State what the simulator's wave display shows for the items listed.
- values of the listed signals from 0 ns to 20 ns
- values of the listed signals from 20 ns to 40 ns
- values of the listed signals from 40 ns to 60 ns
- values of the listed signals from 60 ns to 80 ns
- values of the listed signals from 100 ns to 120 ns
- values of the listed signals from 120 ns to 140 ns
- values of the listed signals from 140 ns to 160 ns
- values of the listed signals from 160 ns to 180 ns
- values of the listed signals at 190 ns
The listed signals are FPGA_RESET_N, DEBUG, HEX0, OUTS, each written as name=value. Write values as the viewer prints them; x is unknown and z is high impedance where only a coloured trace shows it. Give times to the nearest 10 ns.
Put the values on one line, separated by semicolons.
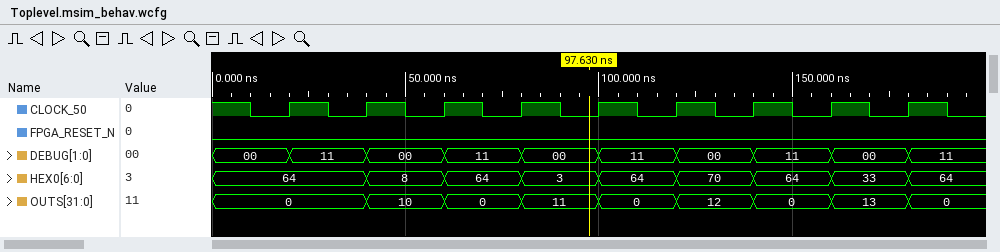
FPGA_RESET_N=0, DEBUG=00, HEX0=64, OUTS=0; FPGA_RESET_N=0, DEBUG=11, HEX0=64, OUTS=0; FPGA_RESET_N=0, DEBUG=00, HEX0=8, OUTS=10; FPGA_RESET_N=0, DEBUG=11, HEX0=64, OUTS=0; FPGA_RESET_N=0, DEBUG=11, HEX0=64, OUTS=0; FPGA_RESET_N=0, DEBUG=00, HEX0=70, OUTS=12; FPGA_RESET_N=0, DEBUG=11, HEX0=64, OUTS=0; FPGA_RESET_N=0, DEBUG=00, HEX0=33, OUTS=13; FPGA_RESET_N=0, DEBUG=11, HEX0=64, OUTS=0
